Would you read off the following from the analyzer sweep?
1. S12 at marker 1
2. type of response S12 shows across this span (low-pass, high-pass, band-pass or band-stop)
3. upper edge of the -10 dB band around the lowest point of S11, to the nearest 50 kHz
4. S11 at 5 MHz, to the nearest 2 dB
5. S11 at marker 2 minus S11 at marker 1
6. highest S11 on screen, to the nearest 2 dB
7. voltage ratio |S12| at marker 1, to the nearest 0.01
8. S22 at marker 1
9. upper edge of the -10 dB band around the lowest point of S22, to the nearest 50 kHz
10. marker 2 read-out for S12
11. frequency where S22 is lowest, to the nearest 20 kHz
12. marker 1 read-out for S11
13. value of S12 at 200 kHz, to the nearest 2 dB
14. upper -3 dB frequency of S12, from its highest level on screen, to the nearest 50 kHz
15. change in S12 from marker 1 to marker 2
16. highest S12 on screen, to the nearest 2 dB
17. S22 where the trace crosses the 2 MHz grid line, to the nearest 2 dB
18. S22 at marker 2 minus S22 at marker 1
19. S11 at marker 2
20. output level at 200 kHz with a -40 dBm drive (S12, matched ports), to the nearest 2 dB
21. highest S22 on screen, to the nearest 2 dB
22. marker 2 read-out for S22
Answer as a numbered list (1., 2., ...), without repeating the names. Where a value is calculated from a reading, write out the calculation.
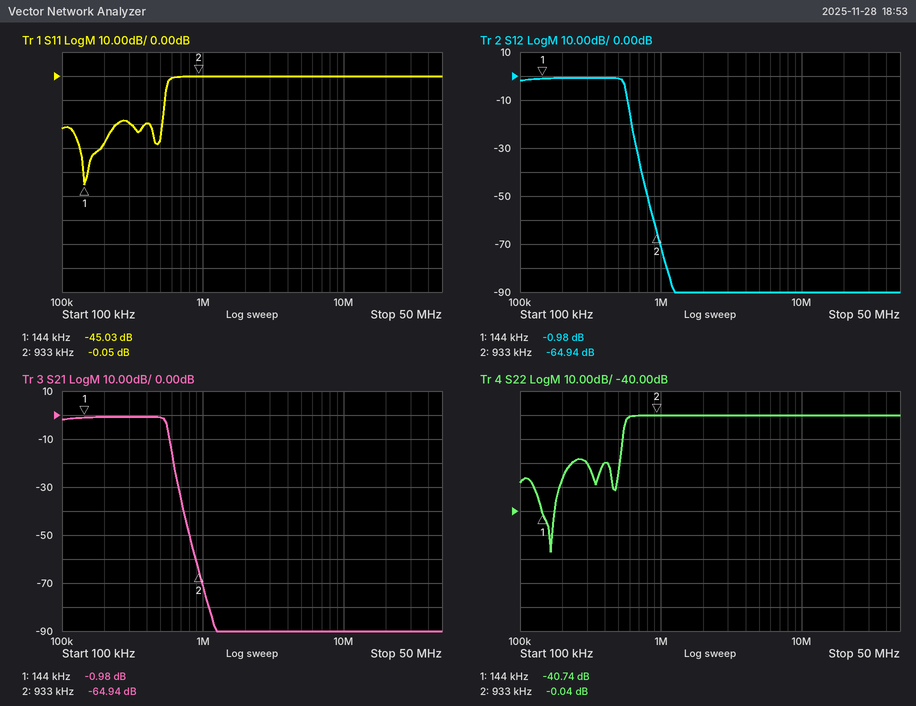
1. -0.98 dB
2. low-pass
3. 550 kHz
4. 0 dB
5. -0.05 − (-45.03) = 44.98 dB
6. 0 dB
7. 10^(-0.98/20) ≈ 0.89
8. -40.74 dB
9. 550 kHz
10. -64.94 dB
11. 160 kHz
12. -45.03 dB
13. 0 dB
14. 550 kHz
15. -64.94 − (-0.98) = -63.96 dB
16. 0 dB
17. 0 dB
18. -0.04 − (-40.74) = 40.70 dB
19. -0.05 dB
20. -40 dBm + (0 dB) = -40 dBm
21. 0 dB
22. -0.04 dB
